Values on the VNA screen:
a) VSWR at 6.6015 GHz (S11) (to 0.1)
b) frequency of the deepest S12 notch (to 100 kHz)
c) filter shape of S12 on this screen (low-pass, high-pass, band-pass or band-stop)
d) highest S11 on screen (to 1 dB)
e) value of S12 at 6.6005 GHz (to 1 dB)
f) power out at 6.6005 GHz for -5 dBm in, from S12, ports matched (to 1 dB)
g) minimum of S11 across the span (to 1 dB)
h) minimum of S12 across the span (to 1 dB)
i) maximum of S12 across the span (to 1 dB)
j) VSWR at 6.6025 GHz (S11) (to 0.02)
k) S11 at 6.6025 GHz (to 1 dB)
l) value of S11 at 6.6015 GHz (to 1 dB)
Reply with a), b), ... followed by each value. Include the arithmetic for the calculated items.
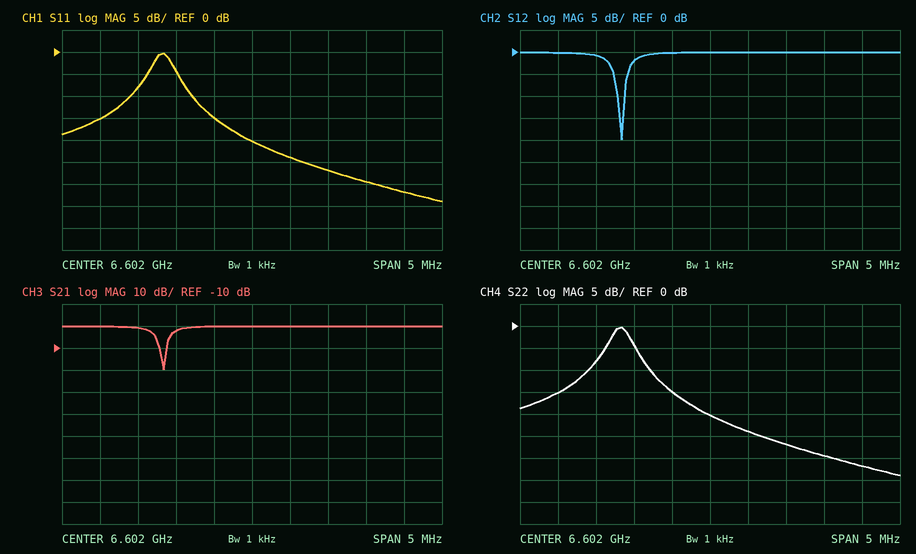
a) |Γ| = 10^(-15/20) = 0.1778; VSWR = (1 + 0.1778)/(1 − 0.1778) ≈ 1.4
b) 6.6008 GHz
c) band-stop
d) 0 dB
e) -1 dB
f) -5 dBm + (-1 dB) = -6 dBm
g) -34 dB
h) -20 dB
i) 0 dB
j) |Γ| = 10^(-24/20) = 0.0631; VSWR = (1 + 0.0631)/(1 − 0.0631) ≈ 1.13, so 1.14 to the nearest 0.02
k) -24 dB
l) -15 dB
